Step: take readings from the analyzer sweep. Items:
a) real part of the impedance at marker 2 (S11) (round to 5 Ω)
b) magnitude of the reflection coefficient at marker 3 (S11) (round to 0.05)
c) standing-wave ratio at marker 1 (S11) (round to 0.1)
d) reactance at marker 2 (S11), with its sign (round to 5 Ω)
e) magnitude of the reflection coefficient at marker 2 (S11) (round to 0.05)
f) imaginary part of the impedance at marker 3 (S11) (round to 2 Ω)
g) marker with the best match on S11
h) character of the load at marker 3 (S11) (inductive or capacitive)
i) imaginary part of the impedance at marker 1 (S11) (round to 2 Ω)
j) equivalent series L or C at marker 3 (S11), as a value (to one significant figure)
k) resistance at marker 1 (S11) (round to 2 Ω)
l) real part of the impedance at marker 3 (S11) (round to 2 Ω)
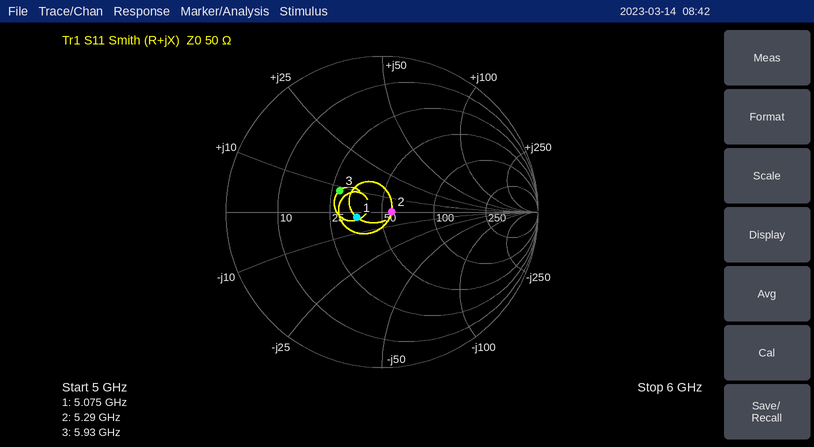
55 Ω
0.30
1.4
0 Ω
0.05
+8 Ω
marker 2
inductive
-2 Ω
200 pH
36 Ω
28 Ω
